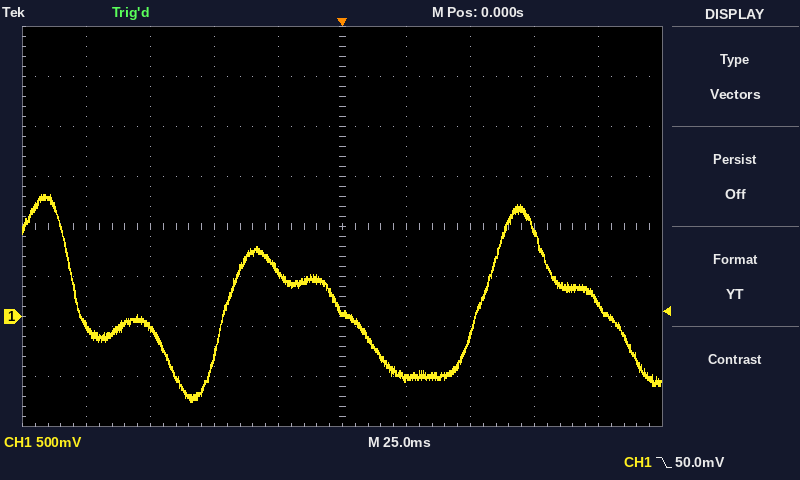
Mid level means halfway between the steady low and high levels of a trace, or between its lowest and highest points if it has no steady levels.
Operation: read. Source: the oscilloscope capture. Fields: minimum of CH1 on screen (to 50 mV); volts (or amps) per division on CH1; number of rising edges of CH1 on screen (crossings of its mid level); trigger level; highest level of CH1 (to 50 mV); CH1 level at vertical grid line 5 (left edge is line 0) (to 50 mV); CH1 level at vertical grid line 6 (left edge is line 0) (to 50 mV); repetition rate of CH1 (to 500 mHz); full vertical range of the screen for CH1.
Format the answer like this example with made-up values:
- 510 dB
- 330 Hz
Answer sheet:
- -850 mV
- 500 mV
- 2
- 50.0 mV
- 1.20 V
- 50 mV
- -600 mV
- 10.0 Hz
- 4 V
